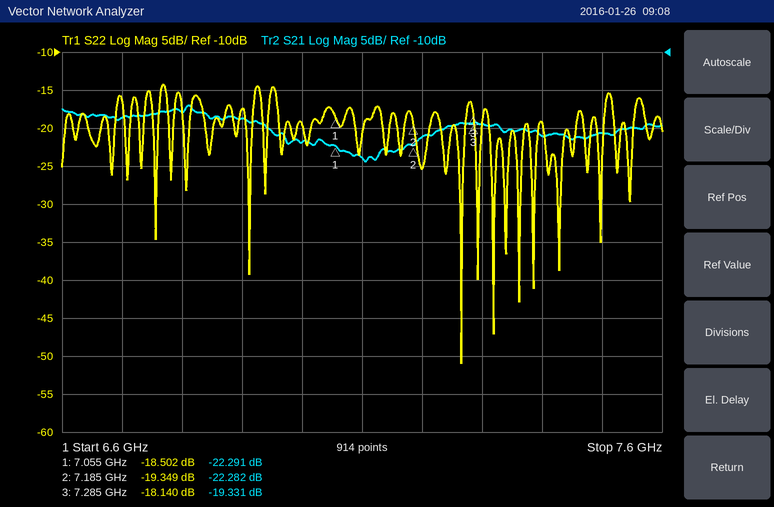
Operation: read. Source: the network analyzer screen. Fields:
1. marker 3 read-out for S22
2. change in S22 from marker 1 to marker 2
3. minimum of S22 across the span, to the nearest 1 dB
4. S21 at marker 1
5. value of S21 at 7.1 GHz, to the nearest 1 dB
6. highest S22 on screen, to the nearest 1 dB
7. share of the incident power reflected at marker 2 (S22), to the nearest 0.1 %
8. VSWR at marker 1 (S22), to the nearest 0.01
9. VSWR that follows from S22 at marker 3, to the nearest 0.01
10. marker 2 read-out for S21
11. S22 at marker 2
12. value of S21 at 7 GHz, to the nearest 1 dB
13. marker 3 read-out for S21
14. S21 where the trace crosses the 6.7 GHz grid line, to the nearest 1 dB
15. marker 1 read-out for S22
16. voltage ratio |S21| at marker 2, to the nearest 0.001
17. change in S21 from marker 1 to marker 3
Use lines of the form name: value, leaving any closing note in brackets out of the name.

marker 3 read-out for S22: -18.140 dB
change in S22 from marker 1 to marker 2: -0.847 dB
minimum of S22 across the span, to the nearest 1 dB: -51 dB
S21 at marker 1: -22.291 dB
value of S21 at 7.1 GHz, to the nearest 1 dB: -24 dB
highest S22 on screen, to the nearest 1 dB: -14 dB
share of the incident power reflected at marker 2 (S22), to the nearest 0.1 %: 1.2 %
VSWR at marker 1 (S22), to the nearest 0.01: 1.27
VSWR that follows from S22 at marker 3, to the nearest 0.01: 1.28
marker 2 read-out for S21: -22.282 dB
S22 at marker 2: -19.349 dB
value of S21 at 7 GHz, to the nearest 1 dB: -22 dB
marker 3 read-out for S21: -19.331 dB
S21 where the trace crosses the 6.7 GHz grid line, to the nearest 1 dB: -19 dB
marker 1 read-out for S22: -18.502 dB
voltage ratio |S21| at marker 2, to the nearest 0.001: 0.077
change in S21 from marker 1 to marker 3: 2.960 dB
